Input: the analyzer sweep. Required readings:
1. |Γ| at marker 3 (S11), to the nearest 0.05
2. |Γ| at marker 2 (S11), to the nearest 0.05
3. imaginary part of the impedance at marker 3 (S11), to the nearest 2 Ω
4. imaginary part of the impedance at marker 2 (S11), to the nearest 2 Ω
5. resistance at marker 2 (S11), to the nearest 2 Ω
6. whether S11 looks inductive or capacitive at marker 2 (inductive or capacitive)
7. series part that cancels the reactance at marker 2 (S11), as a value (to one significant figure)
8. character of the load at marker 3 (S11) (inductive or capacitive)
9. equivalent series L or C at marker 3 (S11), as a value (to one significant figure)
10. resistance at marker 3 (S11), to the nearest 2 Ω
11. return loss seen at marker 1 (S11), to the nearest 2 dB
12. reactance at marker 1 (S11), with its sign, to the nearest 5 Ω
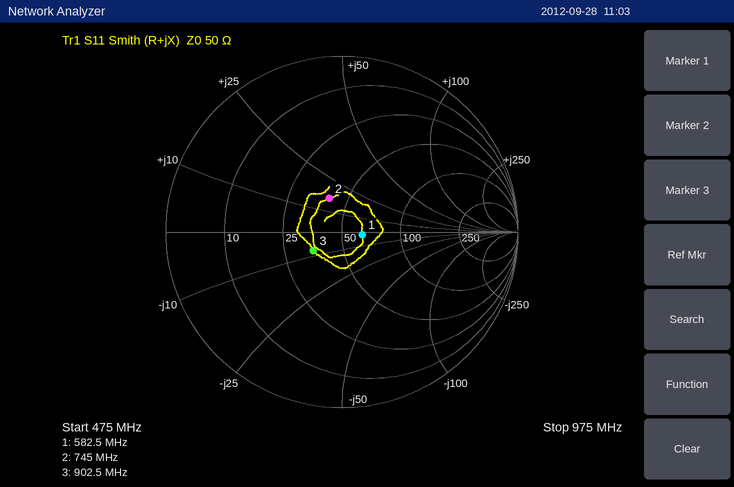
0.20
0.20
-8 Ω
+16 Ω
40 Ω
inductive
10 pF
capacitive
20 pF
36 Ω
18 dB
0 Ω
